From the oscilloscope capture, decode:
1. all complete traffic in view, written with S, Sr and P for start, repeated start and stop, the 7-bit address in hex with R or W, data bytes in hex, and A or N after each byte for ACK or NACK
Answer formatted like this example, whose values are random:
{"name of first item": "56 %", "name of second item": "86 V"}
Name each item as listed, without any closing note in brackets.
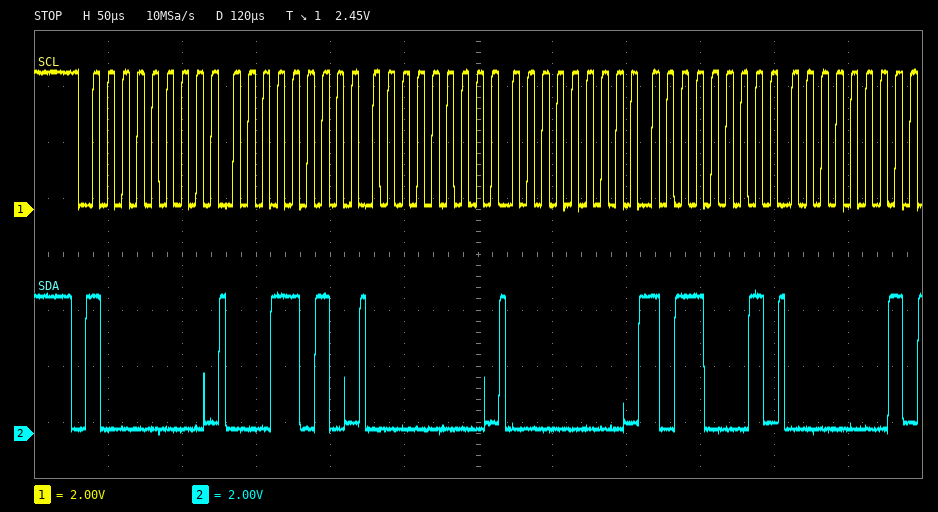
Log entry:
{"all complete traffic in view, written with S, Sr and P for start, repeated start and stop, the 7-bit address in hex with R or W, data bytes in hex, and A or N after each byte for ACK or NACK": "S 40W A 1A A 00 A 00 A B1 A 01 A"}
